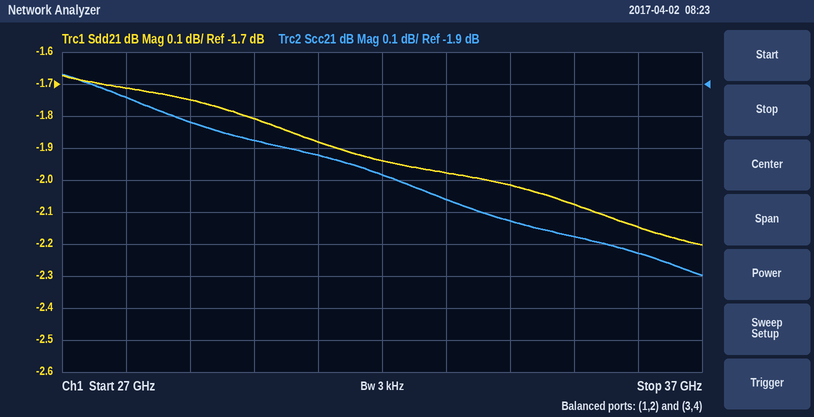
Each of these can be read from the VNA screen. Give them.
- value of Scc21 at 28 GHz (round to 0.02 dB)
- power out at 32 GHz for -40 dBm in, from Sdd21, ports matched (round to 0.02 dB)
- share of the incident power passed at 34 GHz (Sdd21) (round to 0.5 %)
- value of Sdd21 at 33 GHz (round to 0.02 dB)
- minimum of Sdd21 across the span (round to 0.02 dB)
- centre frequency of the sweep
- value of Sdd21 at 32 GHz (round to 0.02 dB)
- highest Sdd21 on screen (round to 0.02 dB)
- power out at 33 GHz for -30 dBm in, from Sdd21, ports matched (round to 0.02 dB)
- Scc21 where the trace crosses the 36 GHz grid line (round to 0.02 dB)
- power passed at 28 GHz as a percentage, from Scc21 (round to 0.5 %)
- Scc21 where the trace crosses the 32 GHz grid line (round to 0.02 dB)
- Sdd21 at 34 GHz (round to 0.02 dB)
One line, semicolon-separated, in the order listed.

-1.94 dB; -41.94 dBm; 63.0 %; -1.98 dB; -2.20 dB; 32 GHz; -1.94 dB; -1.68 dB; -31.98 dBm; -2.42 dB; 64.0 %; -2.18 dB; -2.02 dB
